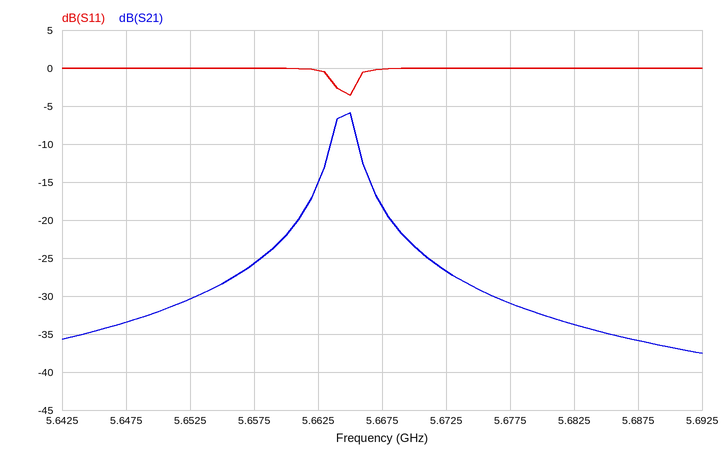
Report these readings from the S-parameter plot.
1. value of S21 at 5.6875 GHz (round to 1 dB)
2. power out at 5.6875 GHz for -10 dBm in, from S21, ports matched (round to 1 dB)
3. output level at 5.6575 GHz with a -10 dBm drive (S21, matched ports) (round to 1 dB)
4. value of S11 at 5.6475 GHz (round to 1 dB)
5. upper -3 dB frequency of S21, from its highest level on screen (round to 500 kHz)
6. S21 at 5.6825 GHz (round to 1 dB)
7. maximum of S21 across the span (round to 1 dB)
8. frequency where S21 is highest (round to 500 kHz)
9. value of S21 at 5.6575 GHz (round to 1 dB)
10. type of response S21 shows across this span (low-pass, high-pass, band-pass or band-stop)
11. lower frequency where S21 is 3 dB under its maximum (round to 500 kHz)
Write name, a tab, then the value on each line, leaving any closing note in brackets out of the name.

value of S21 at 5.6875 GHz	-36 dB
power out at 5.6875 GHz for -10 dBm in, from S21, ports matched	-46 dBm
output level at 5.6575 GHz with a -10 dBm drive (S21, matched ports)	-36 dBm
value of S11 at 5.6475 GHz	0 dB
upper -3 dB frequency of S21, from its highest level on screen	5.6655 GHz
S21 at 5.6825 GHz	-34 dB
maximum of S21 across the span	-6 dB
frequency where S21 is highest	5.6650 GHz
value of S21 at 5.6575 GHz	-26 dB
type of response S21 shows across this span	band-pass
lower frequency where S21 is 3 dB under its maximum	5.6635 GHz
